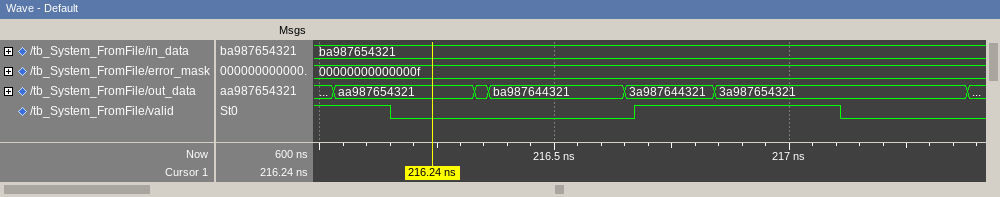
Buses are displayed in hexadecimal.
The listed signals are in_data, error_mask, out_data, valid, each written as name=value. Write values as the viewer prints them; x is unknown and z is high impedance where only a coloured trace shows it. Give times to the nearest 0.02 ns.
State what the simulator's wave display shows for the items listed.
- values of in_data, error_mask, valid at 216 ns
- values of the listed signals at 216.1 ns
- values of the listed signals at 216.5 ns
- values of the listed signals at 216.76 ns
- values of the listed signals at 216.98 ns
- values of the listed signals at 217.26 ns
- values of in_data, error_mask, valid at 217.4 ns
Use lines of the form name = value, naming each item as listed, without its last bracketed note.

values of in_data, error_mask, valid at 216 ns = in_data=ba987654321, error_mask=00000000000000f, valid=1
values of the listed signals at 216.1 ns = in_data=ba987654321, error_mask=00000000000000f, out_data=aa987654321, valid=1
values of the listed signals at 216.5 ns = in_data=ba987654321, error_mask=00000000000000f, out_data=ba987644321, valid=0
values of the listed signals at 216.76 ns = in_data=ba987654321, error_mask=00000000000000f, out_data=3a987644321, valid=1
values of the listed signals at 216.98 ns = in_data=ba987654321, error_mask=00000000000000f, out_data=3a987654321, valid=1
values of the listed signals at 217.26 ns = in_data=ba987654321, error_mask=00000000000000f, out_data=3a987654321, valid=0
values of in_data, error_mask, valid at 217.4 ns = in_data=ba987654321, error_mask=00000000000000f, valid=0
